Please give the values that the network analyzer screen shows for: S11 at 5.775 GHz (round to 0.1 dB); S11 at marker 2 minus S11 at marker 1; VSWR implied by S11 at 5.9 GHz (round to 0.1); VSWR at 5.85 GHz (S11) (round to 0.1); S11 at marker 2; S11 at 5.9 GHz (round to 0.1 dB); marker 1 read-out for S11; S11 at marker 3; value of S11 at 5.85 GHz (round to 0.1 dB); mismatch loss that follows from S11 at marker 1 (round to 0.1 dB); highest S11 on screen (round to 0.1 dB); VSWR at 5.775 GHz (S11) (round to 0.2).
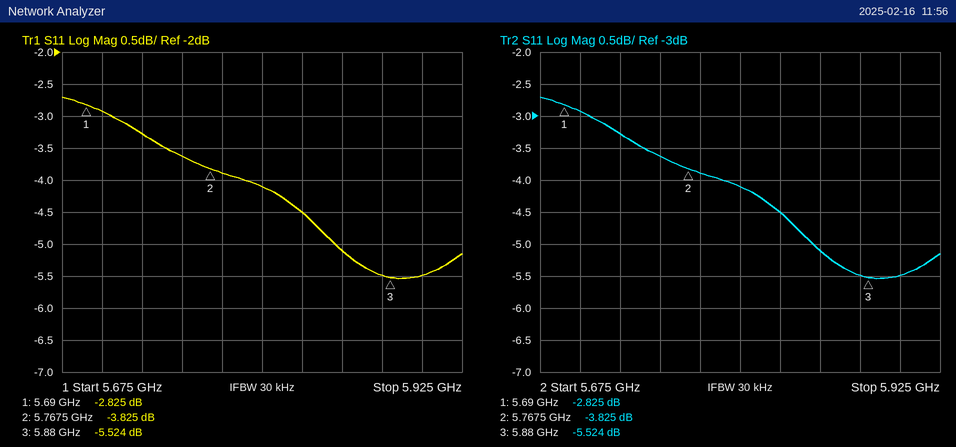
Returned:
-3.9 dB
-1.000 dB
3.3
3.5
-3.825 dB
-5.5 dB
-2.825 dB
-5.524 dB
-5.1 dB
3.2 dB
-2.7 dB
4.6
